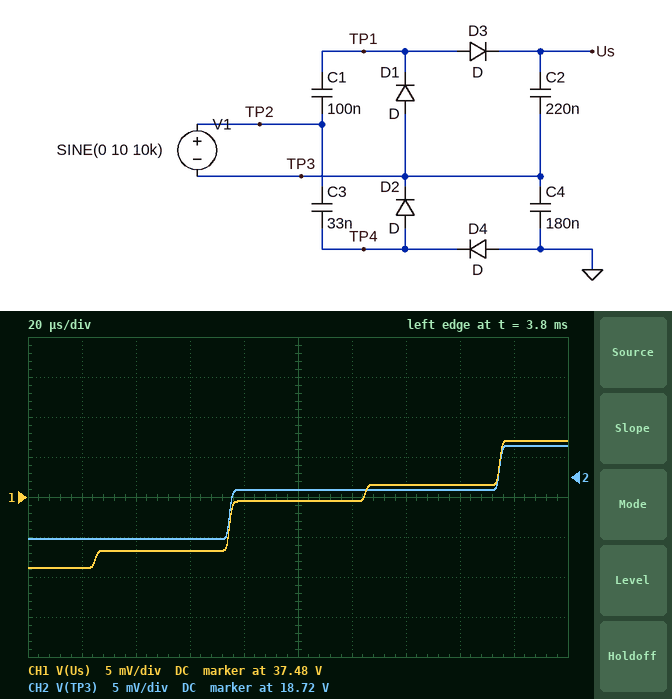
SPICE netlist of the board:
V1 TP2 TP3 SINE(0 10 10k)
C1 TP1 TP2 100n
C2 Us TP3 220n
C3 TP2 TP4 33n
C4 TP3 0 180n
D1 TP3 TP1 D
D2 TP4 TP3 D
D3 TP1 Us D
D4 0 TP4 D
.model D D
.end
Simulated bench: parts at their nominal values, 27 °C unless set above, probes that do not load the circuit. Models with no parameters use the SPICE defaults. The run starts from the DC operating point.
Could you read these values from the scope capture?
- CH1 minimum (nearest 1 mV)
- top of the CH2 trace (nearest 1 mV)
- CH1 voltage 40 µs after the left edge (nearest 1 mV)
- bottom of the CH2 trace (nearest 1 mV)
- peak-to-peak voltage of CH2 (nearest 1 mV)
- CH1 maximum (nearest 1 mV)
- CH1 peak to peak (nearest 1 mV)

37.471 V
18.724 V
37.473 V
18.712 V
12 mV
37.487 V
16 mV
